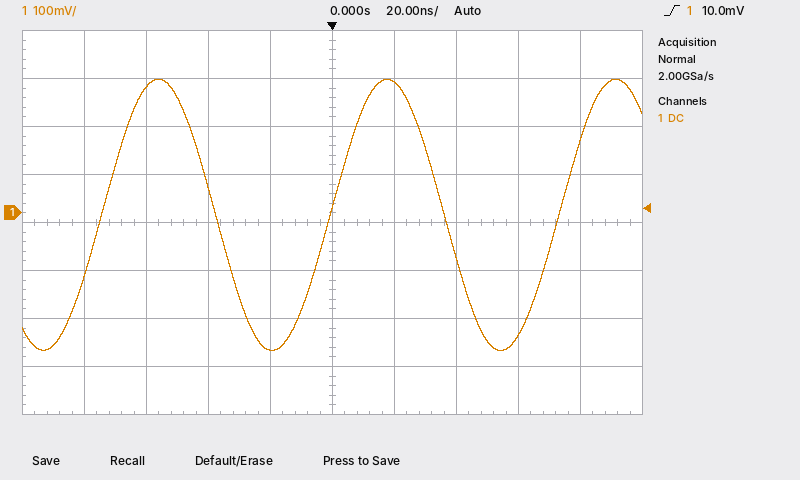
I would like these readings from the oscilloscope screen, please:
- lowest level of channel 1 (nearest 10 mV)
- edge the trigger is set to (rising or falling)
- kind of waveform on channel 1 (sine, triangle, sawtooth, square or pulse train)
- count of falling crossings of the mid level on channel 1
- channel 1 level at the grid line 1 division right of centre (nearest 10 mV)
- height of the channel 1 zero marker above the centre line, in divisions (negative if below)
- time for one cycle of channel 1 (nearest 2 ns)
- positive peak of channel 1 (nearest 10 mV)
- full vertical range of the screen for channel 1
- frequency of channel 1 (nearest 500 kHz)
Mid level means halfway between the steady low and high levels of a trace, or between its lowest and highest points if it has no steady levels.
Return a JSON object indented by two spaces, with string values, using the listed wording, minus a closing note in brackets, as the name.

{
  "lowest level of channel 1": "-290 mV",
  "edge the trigger is set to": "rising",
  "kind of waveform on channel 1": "sine",
  "count of falling crossings of the mid level on channel 1": "2",
  "channel 1 level at the grid line 1 division right of centre": "270 mV",
  "height of the channel 1 zero marker above the centre line, in divisions": "+0.2 div",
  "time for one cycle of channel 1": "74 ns",
  "positive peak of channel 1": "280 mV",
  "full vertical range of the screen for channel 1": "800 mV",
  "frequency of channel 1": "13.5 MHz"
}
